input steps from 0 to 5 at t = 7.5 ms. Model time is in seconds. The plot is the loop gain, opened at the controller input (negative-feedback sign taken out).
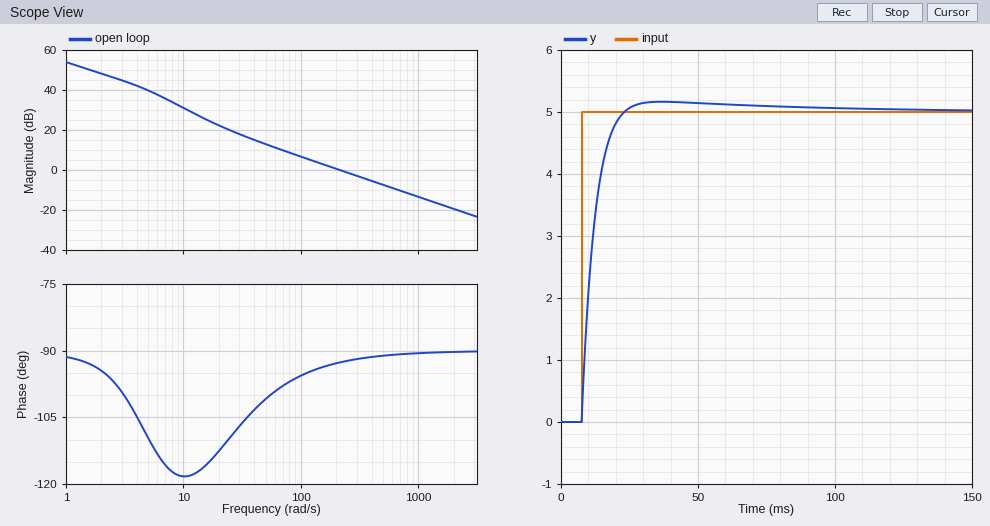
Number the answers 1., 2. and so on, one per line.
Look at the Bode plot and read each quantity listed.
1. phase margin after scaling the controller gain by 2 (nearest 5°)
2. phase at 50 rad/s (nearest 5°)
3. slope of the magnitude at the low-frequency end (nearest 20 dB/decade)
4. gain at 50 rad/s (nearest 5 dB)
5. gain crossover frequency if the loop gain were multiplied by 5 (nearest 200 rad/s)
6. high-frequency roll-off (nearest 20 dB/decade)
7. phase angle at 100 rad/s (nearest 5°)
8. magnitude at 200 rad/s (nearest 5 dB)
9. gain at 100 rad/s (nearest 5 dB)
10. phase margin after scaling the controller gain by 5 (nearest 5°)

1. 90°
2. -100°
3. -20 dB/decade
4. 15 dB
5. 1000 rad/s
6. -20 dB/decade
7. -95°
8. 0 dB
9. 5 dB
10. 90°
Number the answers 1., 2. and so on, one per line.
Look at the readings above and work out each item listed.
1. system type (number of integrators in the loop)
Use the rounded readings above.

1. 1
